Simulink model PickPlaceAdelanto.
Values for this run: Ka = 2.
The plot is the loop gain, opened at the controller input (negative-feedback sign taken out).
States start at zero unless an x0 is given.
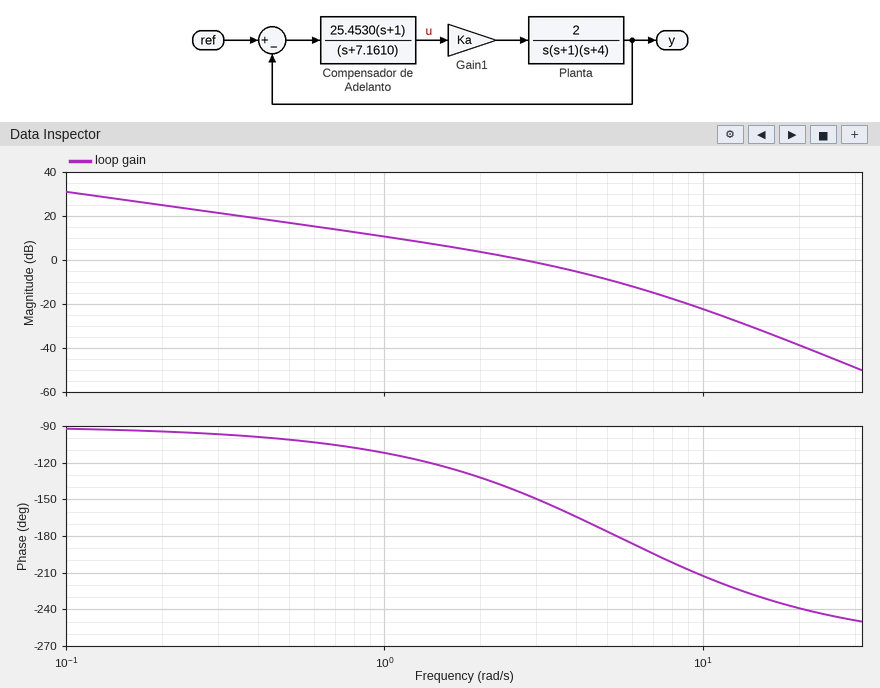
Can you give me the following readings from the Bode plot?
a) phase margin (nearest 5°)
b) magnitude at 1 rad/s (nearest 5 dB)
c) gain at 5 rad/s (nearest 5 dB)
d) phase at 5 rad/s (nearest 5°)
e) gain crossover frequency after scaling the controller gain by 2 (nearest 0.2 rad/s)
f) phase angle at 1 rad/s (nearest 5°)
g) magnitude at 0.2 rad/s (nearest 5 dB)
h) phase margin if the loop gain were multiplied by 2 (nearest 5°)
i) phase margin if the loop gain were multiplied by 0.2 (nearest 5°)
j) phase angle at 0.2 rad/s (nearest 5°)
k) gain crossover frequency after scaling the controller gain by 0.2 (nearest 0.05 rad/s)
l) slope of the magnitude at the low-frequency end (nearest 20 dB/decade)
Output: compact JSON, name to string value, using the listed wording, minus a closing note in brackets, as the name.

{"phase margin": "35°", "magnitude at 1 rad/s": "10 dB", "gain at 5 rad/s": "-10 dB", "phase at 5 rad/s": "-175°", "gain crossover frequency after scaling the controller gain by 2": "4.2 rad/s", "phase angle at 1 rad/s": "-110°", "magnitude at 0.2 rad/s": "25 dB", "phase margin if the loop gain were multiplied by 2": "15°", "phase margin if the loop gain were multiplied by 0.2": "75°", "phase angle at 0.2 rad/s": "-95°", "gain crossover frequency after scaling the controller gain by 0.2": "0.70 rad/s", "slope of the magnitude at the low-frequency end": "-20 dB/decade"}
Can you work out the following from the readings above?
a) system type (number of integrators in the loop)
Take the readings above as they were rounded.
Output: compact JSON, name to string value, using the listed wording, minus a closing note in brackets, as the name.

{"system type": "1"}
